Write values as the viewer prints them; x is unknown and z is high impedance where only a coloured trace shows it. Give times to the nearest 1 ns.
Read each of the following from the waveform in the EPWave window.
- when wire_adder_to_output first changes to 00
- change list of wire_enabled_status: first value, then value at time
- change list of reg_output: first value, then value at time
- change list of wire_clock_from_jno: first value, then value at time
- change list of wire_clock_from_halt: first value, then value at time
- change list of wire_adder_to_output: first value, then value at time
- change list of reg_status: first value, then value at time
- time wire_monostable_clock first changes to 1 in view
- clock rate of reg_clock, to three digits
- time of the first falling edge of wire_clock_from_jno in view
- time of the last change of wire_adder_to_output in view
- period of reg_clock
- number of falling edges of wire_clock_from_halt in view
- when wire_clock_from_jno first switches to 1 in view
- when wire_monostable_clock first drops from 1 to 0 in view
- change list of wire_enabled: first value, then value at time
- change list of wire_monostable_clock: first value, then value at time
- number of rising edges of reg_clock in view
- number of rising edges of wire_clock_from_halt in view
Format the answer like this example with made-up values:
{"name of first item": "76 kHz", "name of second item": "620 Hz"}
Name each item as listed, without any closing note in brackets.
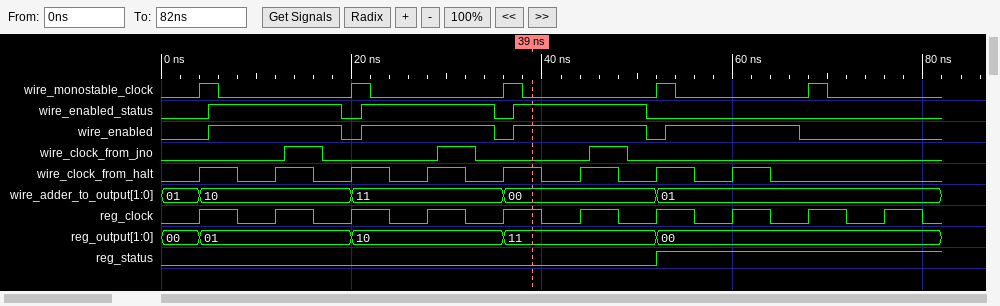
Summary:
{"when wire_adder_to_output first changes to 00": "36 ns", "change list of wire_enabled_status: first value, then value at time": "0, 1 at 5 ns, 0 at 19 ns, 1 at 21 ns, 0 at 35 ns, 1 at 37 ns, 0 at 51 ns", "change list of reg_output: first value, then value at time": "00, 01 at 4 ns, 10 at 20 ns, 11 at 36 ns, 00 at 52 ns", "change list of wire_clock_from_jno: first value, then value at time": "0, 1 at 13 ns, 0 at 17 ns, 1 at 29 ns, 0 at 33 ns, 1 at 45 ns, 0 at 49 ns", "change list of wire_clock_from_halt: first value, then value at time": "0, 1 at 4 ns, 0 at 8 ns, 1 at 12 ns, 0 at 16 ns, 1 at 20 ns, 0 at 24 ns, 1 at 28 ns, 0 at 32 ns, 1 at 36 ns, 0 at 40 ns, 1 at 44 ns, 0 at 48 ns, 1 at 52 ns, 0 at 56 ns, 1 at 60 ns, 0 at 64 ns", "change list of wire_adder_to_output: first value, then value at time": "01, 10 at 4 ns, 11 at 20 ns, 00 at 36 ns, 01 at 52 ns", "change list of reg_status: first value, then value at time": "0, 1 at 52 ns", "time wire_monostable_clock first changes to 1 in view": "4 ns", "clock rate of reg_clock, to three digits": "125 MHz", "time of the first falling edge of wire_clock_from_jno in view": "17 ns", "time of the last change of wire_adder_to_output in view": "52 ns", "period of reg_clock": "8 ns", "number of falling edges of wire_clock_from_halt in view": "8", "when wire_clock_from_jno first switches to 1 in view": "13 ns", "when wire_monostable_clock first drops from 1 to 0 in view": "6 ns", "change list of wire_enabled: first value, then value at time": "0, 1 at 5 ns, 0 at 19 ns, 1 at 21 ns, 0 at 35 ns, 1 at 37 ns, 0 at 51 ns, 1 at 53 ns, 0 at 67 ns", "change list of wire_monostable_clock: first value, then value at time": "0, 1 at 4 ns, 0 at 6 ns, 1 at 20 ns, 0 at 22 ns, 1 at 36 ns, 0 at 38 ns, 1 at 52 ns, 0 at 54 ns, 1 at 68 ns, 0 at 70 ns", "number of rising edges of reg_clock in view": "10", "number of rising edges of wire_clock_from_halt in view": "8"}
